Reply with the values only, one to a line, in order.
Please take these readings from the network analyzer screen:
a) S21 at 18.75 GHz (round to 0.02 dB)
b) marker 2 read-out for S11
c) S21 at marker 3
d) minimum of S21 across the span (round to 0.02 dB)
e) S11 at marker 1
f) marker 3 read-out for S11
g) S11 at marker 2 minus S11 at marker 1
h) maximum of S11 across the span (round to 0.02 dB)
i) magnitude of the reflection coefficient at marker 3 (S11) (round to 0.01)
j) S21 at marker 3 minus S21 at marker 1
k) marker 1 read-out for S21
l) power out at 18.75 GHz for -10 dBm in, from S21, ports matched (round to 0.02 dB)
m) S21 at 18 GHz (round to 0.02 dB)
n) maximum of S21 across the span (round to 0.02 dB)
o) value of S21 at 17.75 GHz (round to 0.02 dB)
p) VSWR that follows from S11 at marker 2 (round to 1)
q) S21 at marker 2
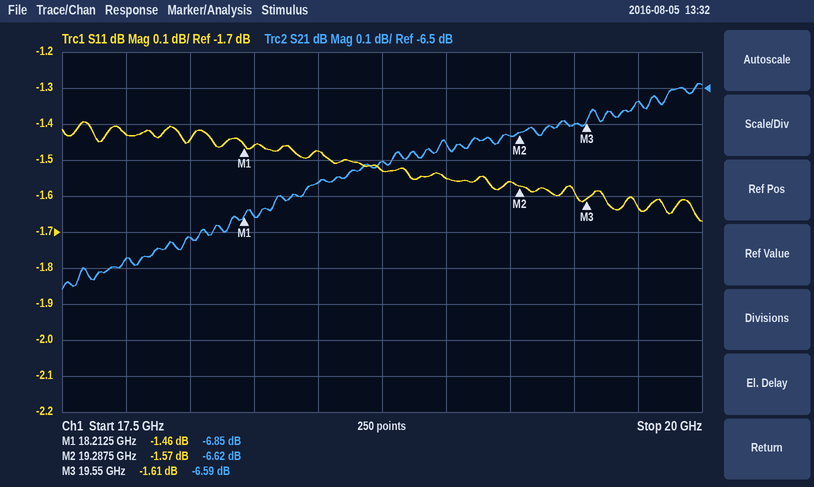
-6.70 dB
-1.57 dB
-6.59 dB
-7.06 dB
-1.46 dB
-1.61 dB
-0.11 dB
-1.40 dB
0.83
0.26 dB
-6.85 dB
-16.70 dBm
-6.92 dB
-6.48 dB
-6.98 dB
11
-6.62 dB
